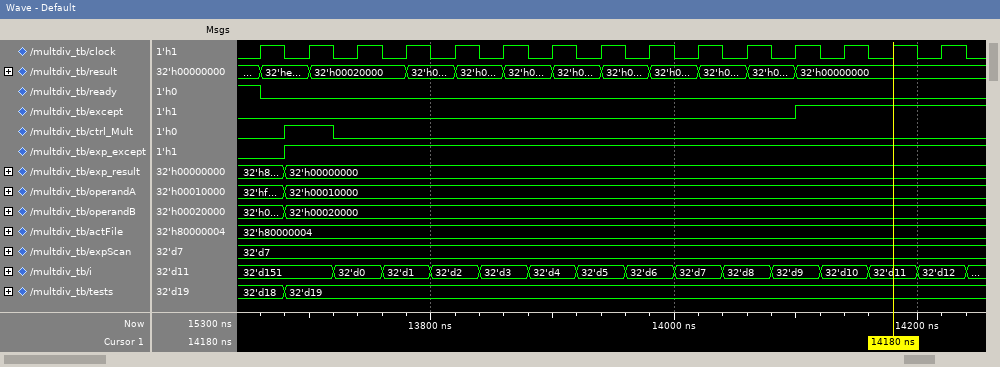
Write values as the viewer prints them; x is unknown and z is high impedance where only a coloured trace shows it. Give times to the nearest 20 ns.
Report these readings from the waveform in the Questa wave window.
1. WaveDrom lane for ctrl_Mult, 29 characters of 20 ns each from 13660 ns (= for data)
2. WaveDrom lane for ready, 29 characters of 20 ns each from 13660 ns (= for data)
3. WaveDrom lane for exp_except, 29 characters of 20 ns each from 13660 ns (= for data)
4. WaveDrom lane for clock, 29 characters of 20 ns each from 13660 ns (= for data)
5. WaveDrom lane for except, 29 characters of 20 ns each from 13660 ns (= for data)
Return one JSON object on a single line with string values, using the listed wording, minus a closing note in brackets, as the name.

{"WaveDrom lane for ctrl_Mult, 29 characters of 20 ns each from 13660 ns": "{name: 'ctrl_Mult', wave: '01.0.........................'}", "WaveDrom lane for ready, 29 characters of 20 ns each from 13660 ns": "{name: 'ready', wave: '0............................'}", "WaveDrom lane for exp_except, 29 characters of 20 ns each from 13660 ns": "{name: 'exp_except', wave: '01...........................'}", "WaveDrom lane for clock, 29 characters of 20 ns each from 13660 ns": "{name: 'clock', wave: '10101010101010101010101010101'}", "WaveDrom lane for except, 29 characters of 20 ns each from 13660 ns": "{name: 'except', wave: '0.....................1......'}"}
